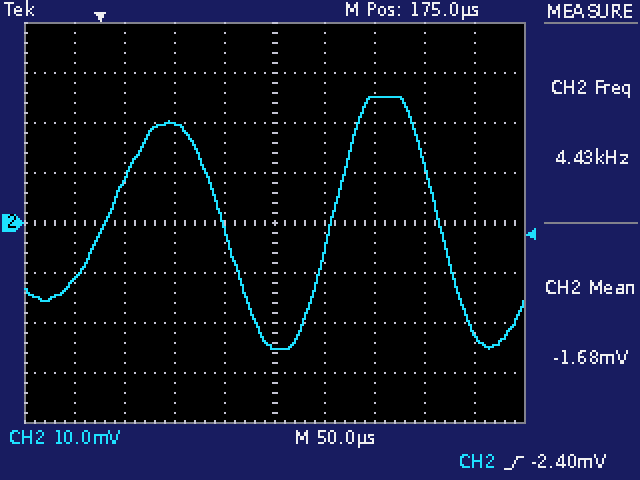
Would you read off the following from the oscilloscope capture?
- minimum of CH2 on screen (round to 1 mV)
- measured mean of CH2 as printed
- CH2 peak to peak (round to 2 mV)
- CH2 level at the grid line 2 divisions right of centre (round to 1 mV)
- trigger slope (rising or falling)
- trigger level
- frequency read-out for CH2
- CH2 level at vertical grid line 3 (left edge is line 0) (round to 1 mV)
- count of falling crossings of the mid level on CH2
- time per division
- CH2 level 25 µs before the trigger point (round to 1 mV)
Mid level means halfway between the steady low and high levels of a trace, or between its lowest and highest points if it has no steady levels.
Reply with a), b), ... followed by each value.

a) -25 mV
b) -1.68 mV
c) 50 mV
d) 25 mV
e) rising
f) -2.40 mV
g) 4.43 kHz
h) 20 mV
i) 2
j) 50 µs
k) -11 mV
